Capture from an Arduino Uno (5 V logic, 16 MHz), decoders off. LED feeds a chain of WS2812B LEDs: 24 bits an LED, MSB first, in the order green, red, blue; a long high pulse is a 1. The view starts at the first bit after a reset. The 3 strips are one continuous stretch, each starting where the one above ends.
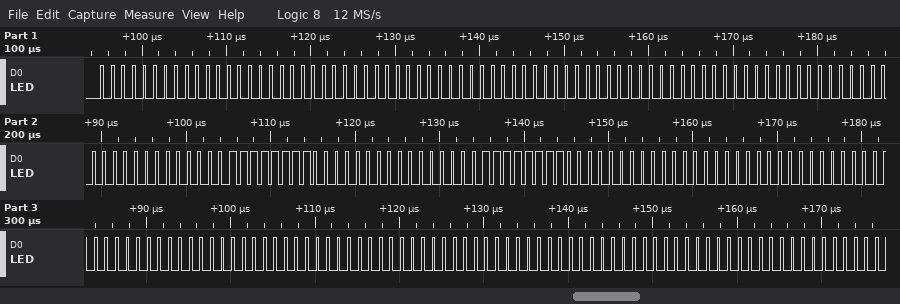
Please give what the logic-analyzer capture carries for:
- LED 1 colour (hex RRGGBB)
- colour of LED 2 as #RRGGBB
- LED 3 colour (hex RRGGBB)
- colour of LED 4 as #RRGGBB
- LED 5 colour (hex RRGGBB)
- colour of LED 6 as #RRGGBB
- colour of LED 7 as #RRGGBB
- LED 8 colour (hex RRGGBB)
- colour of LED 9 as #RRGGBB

#000000
#000000
#000000
#0000FF
#0000FF
#000000
#000000
#000000
#000000
